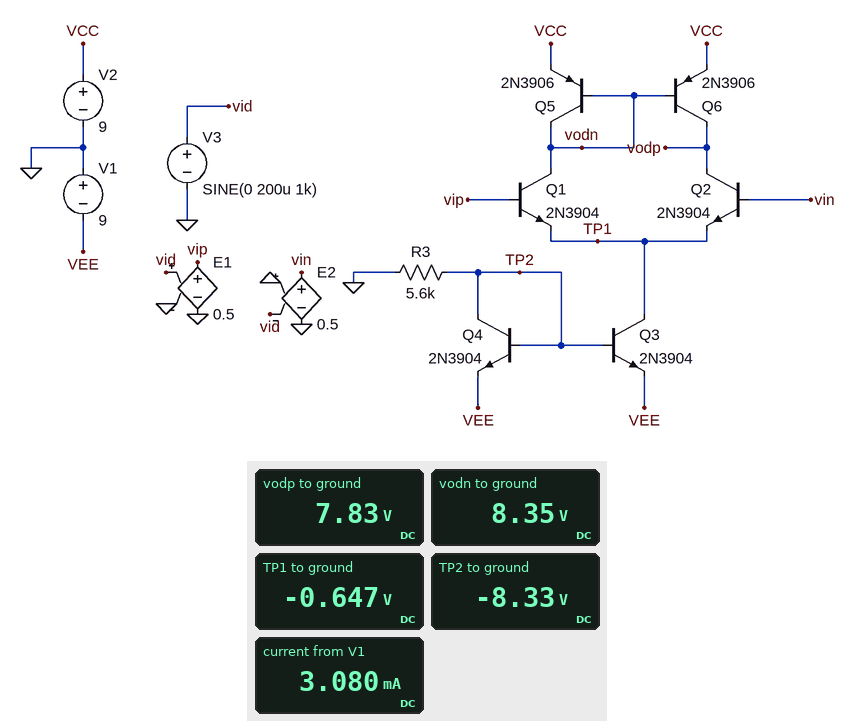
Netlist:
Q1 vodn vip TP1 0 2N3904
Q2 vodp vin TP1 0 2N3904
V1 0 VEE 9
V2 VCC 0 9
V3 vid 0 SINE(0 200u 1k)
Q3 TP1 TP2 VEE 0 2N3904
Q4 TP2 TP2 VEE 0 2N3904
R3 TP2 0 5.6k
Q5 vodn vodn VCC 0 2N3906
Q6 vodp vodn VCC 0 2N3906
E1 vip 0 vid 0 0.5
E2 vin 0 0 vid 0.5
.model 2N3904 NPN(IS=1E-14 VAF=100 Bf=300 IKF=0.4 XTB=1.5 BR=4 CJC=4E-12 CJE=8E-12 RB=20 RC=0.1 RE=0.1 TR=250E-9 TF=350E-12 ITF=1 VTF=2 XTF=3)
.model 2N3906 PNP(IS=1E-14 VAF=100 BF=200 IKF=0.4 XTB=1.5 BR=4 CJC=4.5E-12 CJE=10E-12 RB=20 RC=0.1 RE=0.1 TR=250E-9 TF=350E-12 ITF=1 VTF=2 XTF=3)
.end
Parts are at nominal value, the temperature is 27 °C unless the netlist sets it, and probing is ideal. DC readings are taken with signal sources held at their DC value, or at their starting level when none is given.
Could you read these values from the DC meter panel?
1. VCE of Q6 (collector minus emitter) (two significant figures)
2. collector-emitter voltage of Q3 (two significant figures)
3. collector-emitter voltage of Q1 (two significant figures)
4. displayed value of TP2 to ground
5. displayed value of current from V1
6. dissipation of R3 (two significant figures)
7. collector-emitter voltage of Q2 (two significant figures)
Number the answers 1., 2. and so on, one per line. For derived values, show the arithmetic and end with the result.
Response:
1. 7.83 V - 9 V = -1.2 V
2. -647 mV - (-9 V) = 8.4 V
3. 8.35 V - (-647 mV) = 9.0 V
4. -8.33 V
5. 3.080 mA
6. (0 V - (-8.33 V))^2 / 5.6 kΩ = 12 mW
7. 7.83 V - (-647 mV) = 8.5 V
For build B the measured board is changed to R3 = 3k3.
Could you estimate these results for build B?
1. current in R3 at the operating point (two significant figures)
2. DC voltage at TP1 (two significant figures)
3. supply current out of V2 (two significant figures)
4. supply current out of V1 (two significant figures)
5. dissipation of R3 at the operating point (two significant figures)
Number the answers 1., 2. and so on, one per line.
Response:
1. 2.5 mA
2. -660 mV
3. 2.7 mA
4. 5.2 mA
5. 21 mW
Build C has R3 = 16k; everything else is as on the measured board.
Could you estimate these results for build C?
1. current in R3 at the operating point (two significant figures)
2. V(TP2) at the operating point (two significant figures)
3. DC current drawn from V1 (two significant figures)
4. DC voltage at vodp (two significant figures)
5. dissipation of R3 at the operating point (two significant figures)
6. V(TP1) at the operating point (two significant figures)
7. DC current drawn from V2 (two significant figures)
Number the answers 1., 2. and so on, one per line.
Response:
1. 520 µA
2. -8.4 V
3. 1.1 mA
4. 7.9 V
5. 4.4 mW
6. -620 mV
7. 560 µA
